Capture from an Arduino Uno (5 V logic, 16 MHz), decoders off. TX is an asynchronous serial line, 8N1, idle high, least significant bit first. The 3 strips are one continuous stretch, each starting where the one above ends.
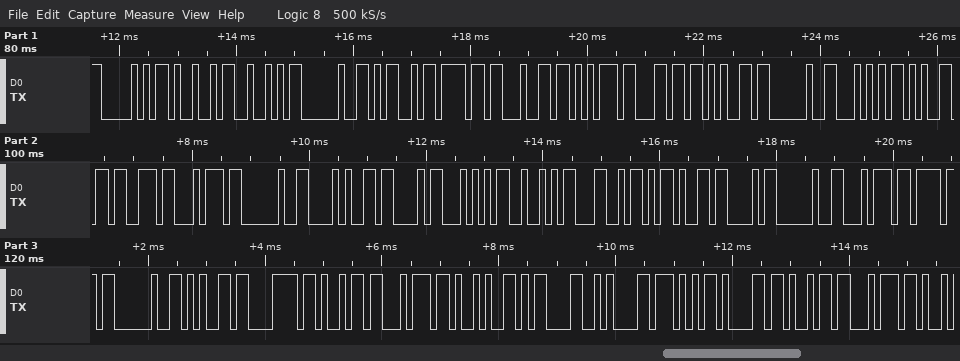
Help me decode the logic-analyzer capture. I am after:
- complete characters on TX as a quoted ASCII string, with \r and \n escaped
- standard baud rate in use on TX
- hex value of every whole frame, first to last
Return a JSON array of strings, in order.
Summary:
["\"PIR Module Test (CTRL-C to exit)\\r\\nWait\"", "9600 baud", "50 49 52 20 4D 6F 64 75 6C 65 20 54 65 73 74 20 28 43 54 52 4C 2D 43 20 74 6F 20 65 78 69 74 29 0D 0A 57 61 69 74"]
